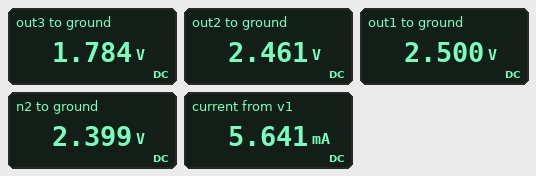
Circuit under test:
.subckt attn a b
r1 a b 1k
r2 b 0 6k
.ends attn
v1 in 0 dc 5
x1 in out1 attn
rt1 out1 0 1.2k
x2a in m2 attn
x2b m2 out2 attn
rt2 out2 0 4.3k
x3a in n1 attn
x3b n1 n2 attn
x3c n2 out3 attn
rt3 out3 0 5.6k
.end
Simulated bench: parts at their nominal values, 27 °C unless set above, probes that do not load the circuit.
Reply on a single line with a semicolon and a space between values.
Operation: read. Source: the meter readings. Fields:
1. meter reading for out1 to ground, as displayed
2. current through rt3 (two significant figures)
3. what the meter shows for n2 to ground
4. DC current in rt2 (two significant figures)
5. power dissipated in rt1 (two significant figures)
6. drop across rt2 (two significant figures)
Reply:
2.500 V; 320 µA; 2.399 V; 570 µA; 5.2 mW; 2.5 V
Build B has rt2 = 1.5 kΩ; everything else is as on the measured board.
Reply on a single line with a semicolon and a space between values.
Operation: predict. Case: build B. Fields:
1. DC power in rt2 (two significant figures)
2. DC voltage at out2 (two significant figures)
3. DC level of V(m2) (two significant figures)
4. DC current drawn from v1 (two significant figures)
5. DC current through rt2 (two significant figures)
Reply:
1.9 mW; 1.7 V; 3.1 V; 6.0 mA; 1.1 mA
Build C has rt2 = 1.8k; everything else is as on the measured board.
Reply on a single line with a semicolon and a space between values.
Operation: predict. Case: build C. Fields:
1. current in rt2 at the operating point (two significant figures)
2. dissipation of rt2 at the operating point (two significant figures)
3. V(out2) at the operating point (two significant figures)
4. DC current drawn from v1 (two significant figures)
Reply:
1.0 mA; 1.9 mW; 1.8 V; 5.9 mA
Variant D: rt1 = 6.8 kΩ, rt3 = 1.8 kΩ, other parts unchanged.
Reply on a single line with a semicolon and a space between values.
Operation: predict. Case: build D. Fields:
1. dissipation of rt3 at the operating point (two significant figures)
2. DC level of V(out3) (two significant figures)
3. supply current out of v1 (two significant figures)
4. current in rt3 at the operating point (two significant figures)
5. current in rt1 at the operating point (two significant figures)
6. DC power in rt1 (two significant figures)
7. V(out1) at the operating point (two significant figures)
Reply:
790 µW; 1.2 V; 4.5 mA; 660 µA; 560 µA; 2.1 mW; 3.8 V
